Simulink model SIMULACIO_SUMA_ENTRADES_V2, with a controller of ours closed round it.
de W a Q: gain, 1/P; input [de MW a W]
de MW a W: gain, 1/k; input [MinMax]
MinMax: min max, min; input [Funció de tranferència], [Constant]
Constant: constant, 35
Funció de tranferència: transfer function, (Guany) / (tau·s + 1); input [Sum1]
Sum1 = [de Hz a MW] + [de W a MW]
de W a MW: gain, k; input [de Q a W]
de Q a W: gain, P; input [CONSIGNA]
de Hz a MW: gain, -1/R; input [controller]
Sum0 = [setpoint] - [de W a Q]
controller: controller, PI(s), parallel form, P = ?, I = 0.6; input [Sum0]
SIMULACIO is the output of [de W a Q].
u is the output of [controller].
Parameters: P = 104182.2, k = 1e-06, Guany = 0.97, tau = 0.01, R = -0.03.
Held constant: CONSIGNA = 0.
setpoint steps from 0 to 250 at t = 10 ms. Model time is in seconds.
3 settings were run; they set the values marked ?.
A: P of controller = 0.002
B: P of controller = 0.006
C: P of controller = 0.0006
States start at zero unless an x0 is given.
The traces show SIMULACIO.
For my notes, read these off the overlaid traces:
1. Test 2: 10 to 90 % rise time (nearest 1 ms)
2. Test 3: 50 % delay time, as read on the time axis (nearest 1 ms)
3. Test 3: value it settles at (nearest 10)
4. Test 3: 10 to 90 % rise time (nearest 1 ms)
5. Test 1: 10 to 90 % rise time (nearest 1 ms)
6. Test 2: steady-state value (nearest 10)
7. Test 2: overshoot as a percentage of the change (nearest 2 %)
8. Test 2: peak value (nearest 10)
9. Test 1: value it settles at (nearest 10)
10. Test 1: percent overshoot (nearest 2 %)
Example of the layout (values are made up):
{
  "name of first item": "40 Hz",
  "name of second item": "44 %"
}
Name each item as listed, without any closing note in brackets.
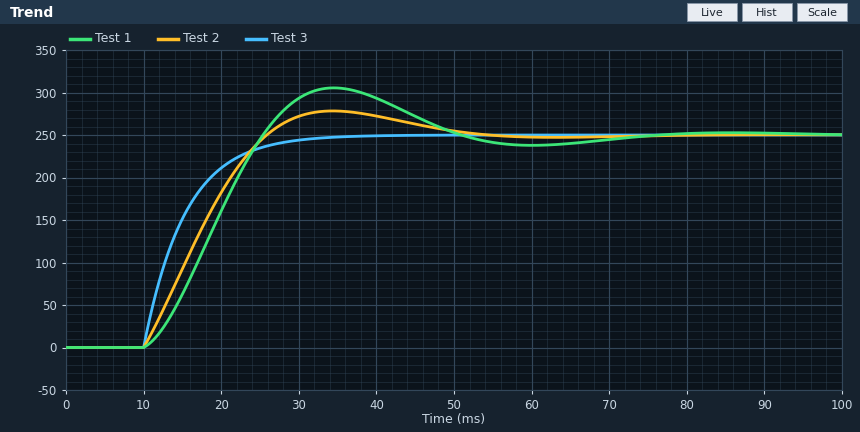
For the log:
{
  "Test 2: 10 to 90 % rise time": "12 ms",
  "Test 3: 50 % delay time, as read on the time axis": "14 ms",
  "Test 3: value it settles at": "250",
  "Test 3: 10 to 90 % rise time": "12 ms",
  "Test 1: 10 to 90 % rise time": "11 ms",
  "Test 2: steady-state value": "250",
  "Test 2: overshoot as a percentage of the change": "12 %",
  "Test 2: peak value": "280",
  "Test 1: value it settles at": "250",
  "Test 1: percent overshoot": "22 %"
}
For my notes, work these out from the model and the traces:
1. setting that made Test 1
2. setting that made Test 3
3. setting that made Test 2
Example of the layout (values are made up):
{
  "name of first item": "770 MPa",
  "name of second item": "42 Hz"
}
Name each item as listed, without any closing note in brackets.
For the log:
{
  "setting that made Test 1": "C",
  "setting that made Test 3": "B",
  "setting that made Test 2": "A"
}
